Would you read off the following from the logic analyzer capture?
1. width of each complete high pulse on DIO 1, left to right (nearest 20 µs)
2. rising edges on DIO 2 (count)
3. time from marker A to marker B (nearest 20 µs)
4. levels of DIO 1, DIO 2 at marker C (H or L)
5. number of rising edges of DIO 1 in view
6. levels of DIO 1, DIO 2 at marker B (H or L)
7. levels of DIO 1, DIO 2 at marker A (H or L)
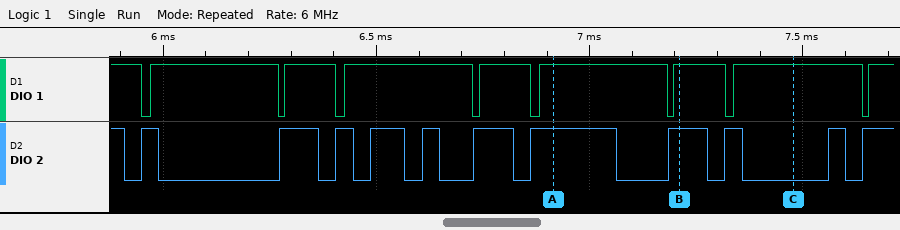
300 µs, 120 µs, 300 µs, 120 µs, 300 µs, 120 µs, 300 µs
11
300 µs
DIO 1=H, DIO 2=L
8
DIO 1=H, DIO 2=H
DIO 1=H, DIO 2=H
